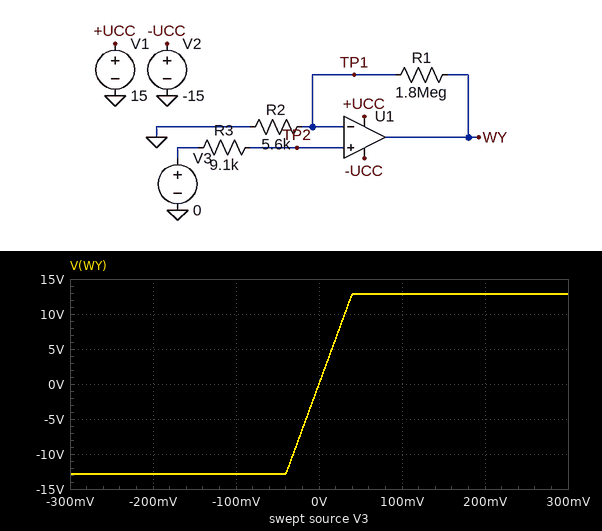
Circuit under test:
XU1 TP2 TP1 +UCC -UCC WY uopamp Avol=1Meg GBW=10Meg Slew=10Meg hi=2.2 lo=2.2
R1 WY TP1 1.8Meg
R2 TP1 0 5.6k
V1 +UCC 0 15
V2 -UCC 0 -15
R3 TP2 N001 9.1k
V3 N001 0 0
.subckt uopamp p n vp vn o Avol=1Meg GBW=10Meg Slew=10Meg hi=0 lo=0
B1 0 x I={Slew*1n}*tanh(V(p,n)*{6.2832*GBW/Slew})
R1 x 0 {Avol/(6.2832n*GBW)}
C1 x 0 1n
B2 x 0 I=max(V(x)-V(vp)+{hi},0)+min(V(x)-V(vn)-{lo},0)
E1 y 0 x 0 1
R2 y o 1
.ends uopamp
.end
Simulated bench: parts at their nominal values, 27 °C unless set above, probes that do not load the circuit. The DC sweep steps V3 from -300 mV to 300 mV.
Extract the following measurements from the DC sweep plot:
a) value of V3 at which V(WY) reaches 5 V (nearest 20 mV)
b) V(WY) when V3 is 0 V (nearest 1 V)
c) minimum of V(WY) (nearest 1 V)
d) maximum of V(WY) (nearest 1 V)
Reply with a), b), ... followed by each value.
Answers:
a) 20 mV
b) 0 V
c) -13 V
d) 13 V
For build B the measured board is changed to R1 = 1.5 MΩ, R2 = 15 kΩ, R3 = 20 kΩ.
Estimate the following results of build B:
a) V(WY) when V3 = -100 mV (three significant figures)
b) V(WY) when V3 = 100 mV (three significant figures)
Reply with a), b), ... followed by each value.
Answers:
a) -10.1 V
b) 10.1 V
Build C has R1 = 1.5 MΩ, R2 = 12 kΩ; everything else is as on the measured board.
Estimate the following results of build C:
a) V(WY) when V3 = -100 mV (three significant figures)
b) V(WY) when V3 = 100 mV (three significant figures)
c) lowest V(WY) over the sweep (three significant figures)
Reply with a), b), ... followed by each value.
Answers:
a) -12.6 V
b) 12.6 V
c) -12.8 V
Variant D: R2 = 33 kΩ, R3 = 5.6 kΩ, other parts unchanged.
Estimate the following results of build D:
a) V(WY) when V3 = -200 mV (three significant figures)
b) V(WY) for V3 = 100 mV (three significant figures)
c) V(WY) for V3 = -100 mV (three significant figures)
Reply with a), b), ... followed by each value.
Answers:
a) -11.1 V
b) 5.55 V
c) -5.55 V
